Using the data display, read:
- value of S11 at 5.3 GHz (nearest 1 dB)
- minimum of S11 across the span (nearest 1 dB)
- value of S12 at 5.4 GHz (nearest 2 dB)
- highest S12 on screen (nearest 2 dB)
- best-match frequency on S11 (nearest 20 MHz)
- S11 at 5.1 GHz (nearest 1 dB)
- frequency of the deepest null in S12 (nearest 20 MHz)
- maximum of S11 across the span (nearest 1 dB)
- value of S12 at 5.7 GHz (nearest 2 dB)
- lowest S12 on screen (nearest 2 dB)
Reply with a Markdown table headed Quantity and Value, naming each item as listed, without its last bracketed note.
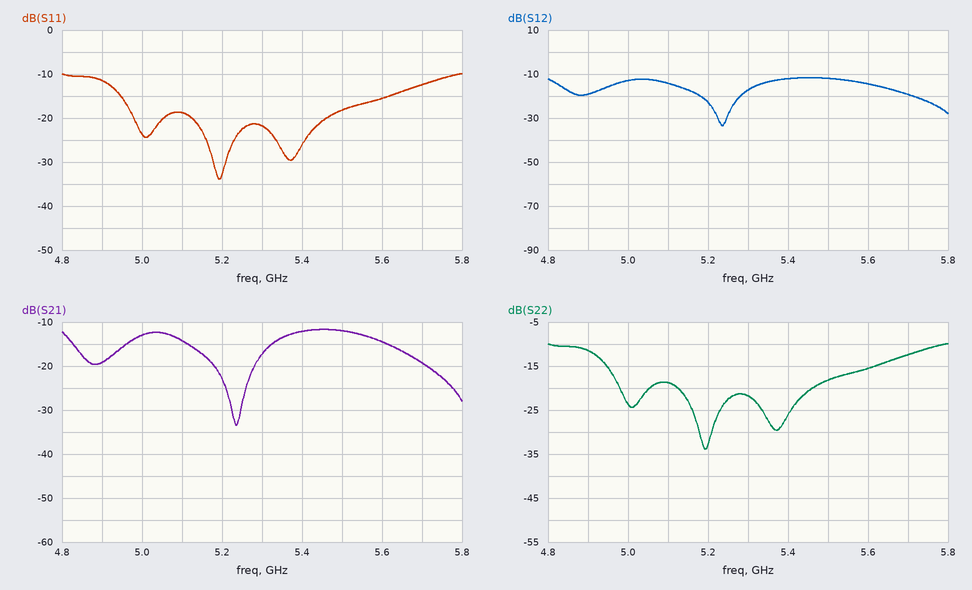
| Quantity | Value |
|---|---|
| value of S11 at 5.3 GHz | -22 dB |
| minimum of S11 across the span | -34 dB |
| value of S12 at 5.4 GHz | -12 dB |
| highest S12 on screen | -12 dB |
| best-match frequency on S11 | 5.20 GHz |
| S11 at 5.1 GHz | -19 dB |
| frequency of the deepest null in S12 | 5.24 GHz |
| maximum of S11 across the span | -10 dB |
| value of S12 at 5.7 GHz | -20 dB |
| lowest S12 on screen | -34 dB |
